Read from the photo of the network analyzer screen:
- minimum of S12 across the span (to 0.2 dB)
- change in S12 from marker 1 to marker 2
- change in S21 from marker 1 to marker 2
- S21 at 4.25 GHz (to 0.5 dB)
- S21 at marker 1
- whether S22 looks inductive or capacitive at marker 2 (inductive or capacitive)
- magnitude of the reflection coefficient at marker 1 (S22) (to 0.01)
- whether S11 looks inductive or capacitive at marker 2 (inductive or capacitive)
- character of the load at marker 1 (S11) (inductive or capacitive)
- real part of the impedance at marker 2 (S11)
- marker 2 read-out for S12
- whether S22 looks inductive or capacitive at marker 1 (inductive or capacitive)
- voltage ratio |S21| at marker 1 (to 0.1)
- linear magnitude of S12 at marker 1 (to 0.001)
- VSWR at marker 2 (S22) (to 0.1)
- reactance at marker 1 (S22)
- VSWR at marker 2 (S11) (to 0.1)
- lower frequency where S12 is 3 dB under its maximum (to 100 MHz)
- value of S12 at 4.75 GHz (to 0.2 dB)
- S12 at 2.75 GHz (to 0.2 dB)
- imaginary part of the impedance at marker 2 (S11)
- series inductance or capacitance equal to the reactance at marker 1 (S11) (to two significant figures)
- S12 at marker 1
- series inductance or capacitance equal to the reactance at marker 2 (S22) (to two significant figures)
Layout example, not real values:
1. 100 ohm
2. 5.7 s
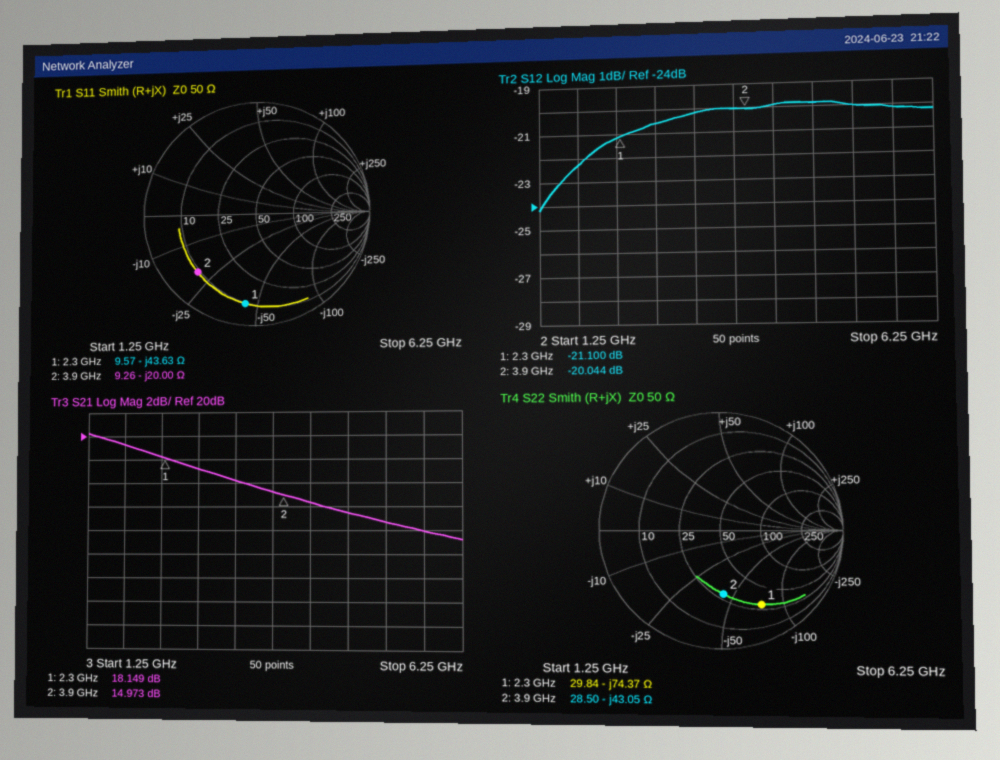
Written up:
1. -24.2 dB
2. 1.056 dB
3. -3.176 dB
4. 14.5 dB
5. 18.149 dB
6. capacitive
7. 0.71
8. capacitive
9. capacitive
10. 9.26 Ω
11. -20.044 dB
12. capacitive
13. 8.1
14. 0.088
15. 3.3
16. -74.37 Ω
17. 6.3
18. 1.6 GHz
19. -19.8 dB
20. -20.6 dB
21. -20.00 Ω
22. 1.6 pF
23. -21.100 dB
24. 950 fF
